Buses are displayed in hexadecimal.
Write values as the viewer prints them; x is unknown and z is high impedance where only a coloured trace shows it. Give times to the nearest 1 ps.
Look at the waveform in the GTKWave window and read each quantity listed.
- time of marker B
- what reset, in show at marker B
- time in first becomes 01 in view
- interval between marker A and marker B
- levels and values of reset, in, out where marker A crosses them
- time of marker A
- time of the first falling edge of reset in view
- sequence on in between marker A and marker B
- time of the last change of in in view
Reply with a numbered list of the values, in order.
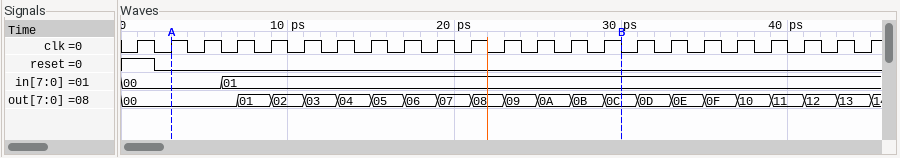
1. 30 ps
2. reset=0, in=01
3. 6 ps
4. 27 ps
5. reset=0, in=00, out=00
6. 3 ps
7. 2 ps
8. 00, 01
9. 6 ps
